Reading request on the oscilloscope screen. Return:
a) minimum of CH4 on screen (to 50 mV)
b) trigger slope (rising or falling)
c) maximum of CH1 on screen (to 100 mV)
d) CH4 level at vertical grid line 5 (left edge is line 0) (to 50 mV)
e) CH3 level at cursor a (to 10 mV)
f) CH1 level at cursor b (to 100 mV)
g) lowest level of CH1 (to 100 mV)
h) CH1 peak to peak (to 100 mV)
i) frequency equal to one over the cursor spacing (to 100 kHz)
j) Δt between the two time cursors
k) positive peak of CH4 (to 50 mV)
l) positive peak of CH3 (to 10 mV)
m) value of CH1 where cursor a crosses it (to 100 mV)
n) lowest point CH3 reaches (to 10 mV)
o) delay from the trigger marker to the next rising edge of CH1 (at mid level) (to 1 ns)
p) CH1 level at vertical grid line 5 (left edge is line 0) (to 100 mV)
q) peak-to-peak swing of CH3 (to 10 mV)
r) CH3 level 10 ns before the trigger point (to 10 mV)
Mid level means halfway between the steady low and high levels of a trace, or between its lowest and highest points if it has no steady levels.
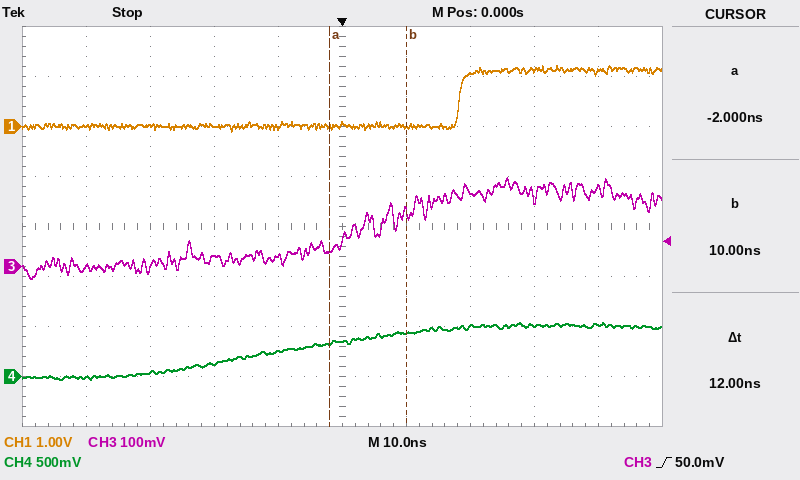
-50 mV
rising
1.2 V
350 mV
30 mV
0.0 V
-100 mV
1.3 V
83.3 MHz
12 ns
550 mV
180 mV
0.0 V
-20 mV
18 ns
0.0 V
200 mV
20 mV
